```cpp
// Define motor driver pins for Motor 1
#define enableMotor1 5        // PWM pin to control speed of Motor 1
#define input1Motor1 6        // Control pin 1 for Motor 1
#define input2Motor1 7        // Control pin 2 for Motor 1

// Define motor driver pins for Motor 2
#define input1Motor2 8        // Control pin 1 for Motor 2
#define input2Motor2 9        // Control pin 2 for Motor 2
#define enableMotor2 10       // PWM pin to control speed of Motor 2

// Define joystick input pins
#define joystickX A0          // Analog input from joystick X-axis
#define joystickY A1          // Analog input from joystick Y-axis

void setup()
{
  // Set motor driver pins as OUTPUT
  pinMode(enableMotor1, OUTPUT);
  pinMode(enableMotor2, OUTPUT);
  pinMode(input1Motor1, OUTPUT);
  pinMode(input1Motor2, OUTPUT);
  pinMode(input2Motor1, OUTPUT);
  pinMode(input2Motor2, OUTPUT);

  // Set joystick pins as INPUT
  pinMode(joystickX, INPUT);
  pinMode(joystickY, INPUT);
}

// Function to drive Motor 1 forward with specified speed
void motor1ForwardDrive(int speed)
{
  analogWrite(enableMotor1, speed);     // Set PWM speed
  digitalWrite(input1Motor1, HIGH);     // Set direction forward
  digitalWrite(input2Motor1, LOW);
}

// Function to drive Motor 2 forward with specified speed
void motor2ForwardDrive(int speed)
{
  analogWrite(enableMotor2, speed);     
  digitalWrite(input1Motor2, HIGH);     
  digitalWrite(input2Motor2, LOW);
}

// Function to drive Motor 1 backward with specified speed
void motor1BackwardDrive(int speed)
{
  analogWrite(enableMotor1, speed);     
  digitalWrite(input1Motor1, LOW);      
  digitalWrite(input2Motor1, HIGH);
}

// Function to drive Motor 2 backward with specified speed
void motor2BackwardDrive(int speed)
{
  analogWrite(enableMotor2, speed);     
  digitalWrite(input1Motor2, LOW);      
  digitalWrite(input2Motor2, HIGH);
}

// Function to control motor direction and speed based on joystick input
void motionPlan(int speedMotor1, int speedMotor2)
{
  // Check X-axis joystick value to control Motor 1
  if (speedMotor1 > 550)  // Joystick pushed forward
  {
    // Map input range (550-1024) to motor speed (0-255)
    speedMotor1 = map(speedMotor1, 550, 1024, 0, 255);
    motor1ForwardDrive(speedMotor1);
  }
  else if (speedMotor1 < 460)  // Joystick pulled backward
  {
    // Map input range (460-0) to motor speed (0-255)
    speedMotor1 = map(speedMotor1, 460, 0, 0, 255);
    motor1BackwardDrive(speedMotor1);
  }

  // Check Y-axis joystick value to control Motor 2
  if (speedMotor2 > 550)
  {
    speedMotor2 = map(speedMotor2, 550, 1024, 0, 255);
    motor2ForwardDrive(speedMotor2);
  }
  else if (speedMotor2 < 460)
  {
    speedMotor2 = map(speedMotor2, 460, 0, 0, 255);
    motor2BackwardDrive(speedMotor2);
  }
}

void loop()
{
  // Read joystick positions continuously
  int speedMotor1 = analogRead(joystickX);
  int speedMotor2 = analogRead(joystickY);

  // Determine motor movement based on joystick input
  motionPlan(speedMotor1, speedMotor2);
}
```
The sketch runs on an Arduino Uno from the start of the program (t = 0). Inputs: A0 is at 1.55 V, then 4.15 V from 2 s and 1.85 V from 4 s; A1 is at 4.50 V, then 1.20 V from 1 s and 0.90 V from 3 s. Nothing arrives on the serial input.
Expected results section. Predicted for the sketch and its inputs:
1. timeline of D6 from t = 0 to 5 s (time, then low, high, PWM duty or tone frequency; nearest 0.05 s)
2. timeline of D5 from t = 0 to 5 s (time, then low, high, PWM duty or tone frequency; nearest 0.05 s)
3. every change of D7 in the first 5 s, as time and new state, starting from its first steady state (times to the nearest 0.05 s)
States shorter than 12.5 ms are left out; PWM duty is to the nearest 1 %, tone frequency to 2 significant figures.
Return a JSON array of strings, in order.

["0 s low; 2 s high; 4 s low", "0 s PWM 31 %; 2 s PWM 63 %; 4 s PWM 18 %", "0 s high; 2 s low; 4 s high"]
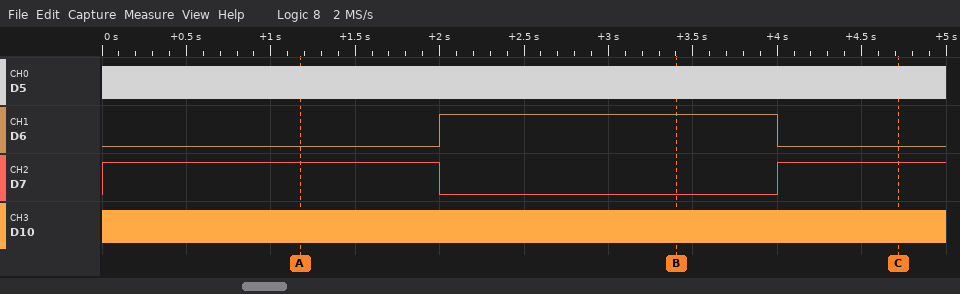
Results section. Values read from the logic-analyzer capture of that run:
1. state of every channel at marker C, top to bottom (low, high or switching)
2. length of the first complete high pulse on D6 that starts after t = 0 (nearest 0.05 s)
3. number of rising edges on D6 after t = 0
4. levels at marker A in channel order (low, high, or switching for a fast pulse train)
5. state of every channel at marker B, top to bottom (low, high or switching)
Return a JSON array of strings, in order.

["D5 switching, D6 low, D7 high, D10 switching", "2.00 s", "1", "D5 switching, D6 low, D7 high, D10 switching", "D5 switching, D6 high, D7 low, D10 switching"]
